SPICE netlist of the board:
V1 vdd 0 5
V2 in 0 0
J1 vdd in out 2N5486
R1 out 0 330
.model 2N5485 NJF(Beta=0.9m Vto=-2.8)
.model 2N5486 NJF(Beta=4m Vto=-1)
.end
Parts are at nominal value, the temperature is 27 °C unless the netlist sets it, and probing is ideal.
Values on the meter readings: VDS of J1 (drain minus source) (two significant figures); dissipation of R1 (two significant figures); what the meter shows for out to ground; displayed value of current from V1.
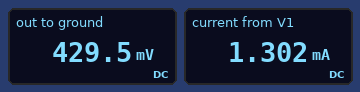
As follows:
4.6 V
560 µW
429.5 mV
1.302 mA
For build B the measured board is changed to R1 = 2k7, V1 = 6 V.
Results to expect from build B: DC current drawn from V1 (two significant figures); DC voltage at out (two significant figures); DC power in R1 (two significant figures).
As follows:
270 µA
740 mV
200 µW
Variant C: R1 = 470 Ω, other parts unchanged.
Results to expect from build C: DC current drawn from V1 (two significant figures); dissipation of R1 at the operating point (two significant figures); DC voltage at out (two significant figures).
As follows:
1.0 mA
510 µW
490 mV
